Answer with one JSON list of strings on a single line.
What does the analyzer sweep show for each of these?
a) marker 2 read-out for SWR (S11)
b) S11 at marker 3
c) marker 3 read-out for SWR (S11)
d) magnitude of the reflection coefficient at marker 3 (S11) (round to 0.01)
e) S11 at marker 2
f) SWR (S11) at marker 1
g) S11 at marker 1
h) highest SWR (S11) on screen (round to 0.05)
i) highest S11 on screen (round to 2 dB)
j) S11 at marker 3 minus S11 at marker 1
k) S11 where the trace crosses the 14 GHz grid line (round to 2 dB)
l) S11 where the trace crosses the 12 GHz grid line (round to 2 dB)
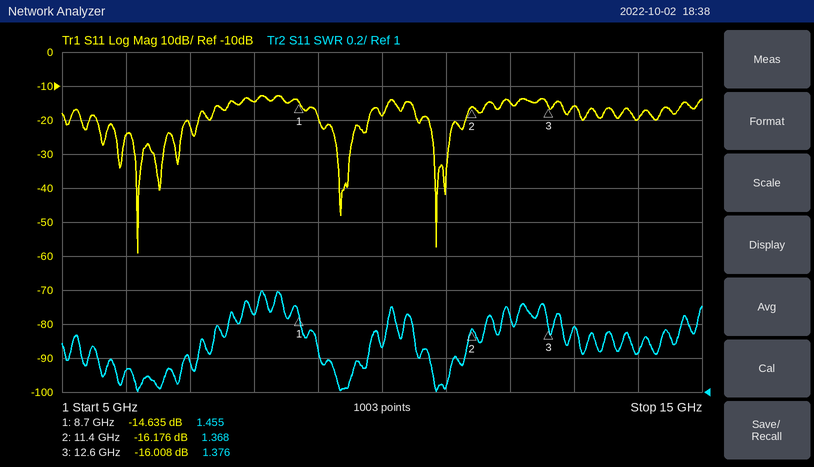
["1.368", "-16.008 dB", "1.376", "0.16", "-16.176 dB", "1.455", "-14.635 dB", "1.60", "-12 dB", "-1.373 dB", "-20 dB", "-14 dB"]
